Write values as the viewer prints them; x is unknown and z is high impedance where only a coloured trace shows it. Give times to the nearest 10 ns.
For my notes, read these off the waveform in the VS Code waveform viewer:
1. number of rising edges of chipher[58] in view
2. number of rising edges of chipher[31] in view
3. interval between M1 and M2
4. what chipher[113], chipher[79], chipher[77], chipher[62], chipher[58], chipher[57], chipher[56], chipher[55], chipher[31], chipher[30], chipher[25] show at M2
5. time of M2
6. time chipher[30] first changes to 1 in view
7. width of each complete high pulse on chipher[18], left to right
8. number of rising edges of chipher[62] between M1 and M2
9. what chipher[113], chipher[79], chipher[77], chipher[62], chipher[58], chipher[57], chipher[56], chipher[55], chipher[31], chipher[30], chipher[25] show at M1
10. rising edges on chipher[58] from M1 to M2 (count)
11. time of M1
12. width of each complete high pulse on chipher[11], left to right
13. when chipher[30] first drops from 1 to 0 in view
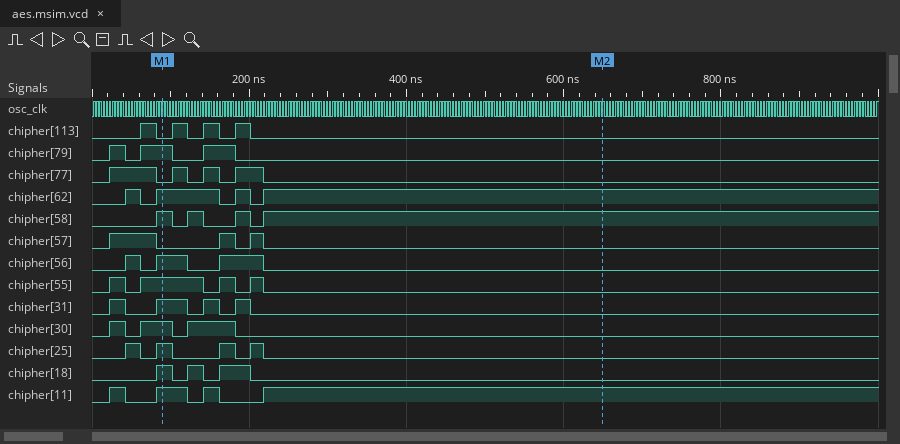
4
4
560 ns
chipher[113]=0, chipher[79]=0, chipher[77]=0, chipher[62]=1, chipher[58]=1, chipher[57]=0, chipher[56]=0, chipher[55]=0, chipher[31]=0, chipher[30]=0, chipher[25]=0
650 ns
20 ns
20 ns, 20 ns, 40 ns
2
chipher[113]=0, chipher[79]=1, chipher[77]=0, chipher[62]=1, chipher[58]=1, chipher[57]=0, chipher[56]=1, chipher[55]=1, chipher[31]=1, chipher[30]=1, chipher[25]=1
3
90 ns
20 ns, 40 ns, 20 ns
40 ns
